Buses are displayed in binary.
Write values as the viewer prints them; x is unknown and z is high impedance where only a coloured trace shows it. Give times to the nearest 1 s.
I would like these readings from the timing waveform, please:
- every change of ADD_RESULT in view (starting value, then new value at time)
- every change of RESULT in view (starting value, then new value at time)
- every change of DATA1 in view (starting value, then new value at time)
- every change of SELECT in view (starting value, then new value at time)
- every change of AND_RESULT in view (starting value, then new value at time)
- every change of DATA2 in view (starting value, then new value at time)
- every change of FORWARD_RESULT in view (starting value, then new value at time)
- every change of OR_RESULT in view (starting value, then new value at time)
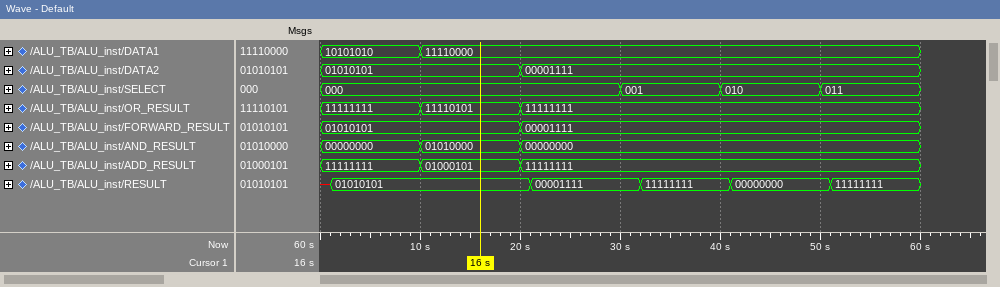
11111111, 01000101 at 10 s, 11111111 at 20 s
x, 01010101 at 1 s, 00001111 at 21 s, 11111111 at 32 s, 00000000 at 41 s, 11111111 at 51 s
10101010, 11110000 at 10 s
000, 001 at 30 s, 010 at 40 s, 011 at 50 s
00000000, 01010000 at 10 s, 00000000 at 20 s
01010101, 00001111 at 20 s
01010101, 00001111 at 20 s
11111111, 11110101 at 10 s, 11111111 at 20 s
